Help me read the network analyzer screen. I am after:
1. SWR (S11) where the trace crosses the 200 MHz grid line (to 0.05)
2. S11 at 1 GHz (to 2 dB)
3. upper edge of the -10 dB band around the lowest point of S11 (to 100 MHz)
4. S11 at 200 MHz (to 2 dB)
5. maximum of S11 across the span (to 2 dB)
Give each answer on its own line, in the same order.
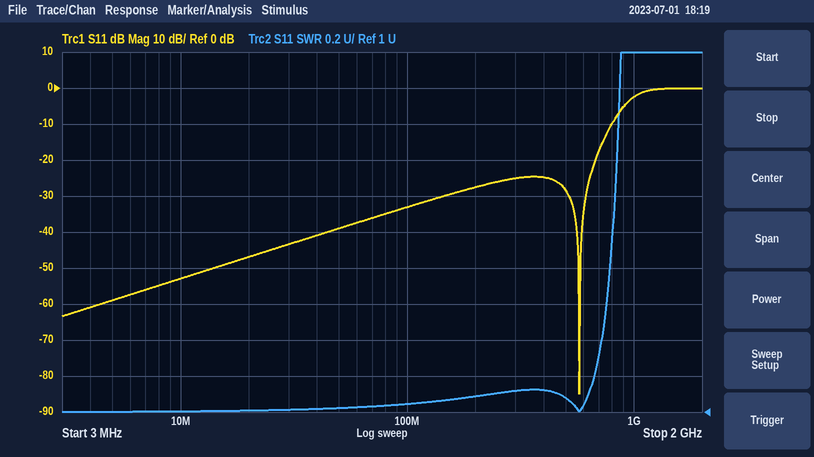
1.10
-2 dB
800 MHz
-28 dB
0 dB
